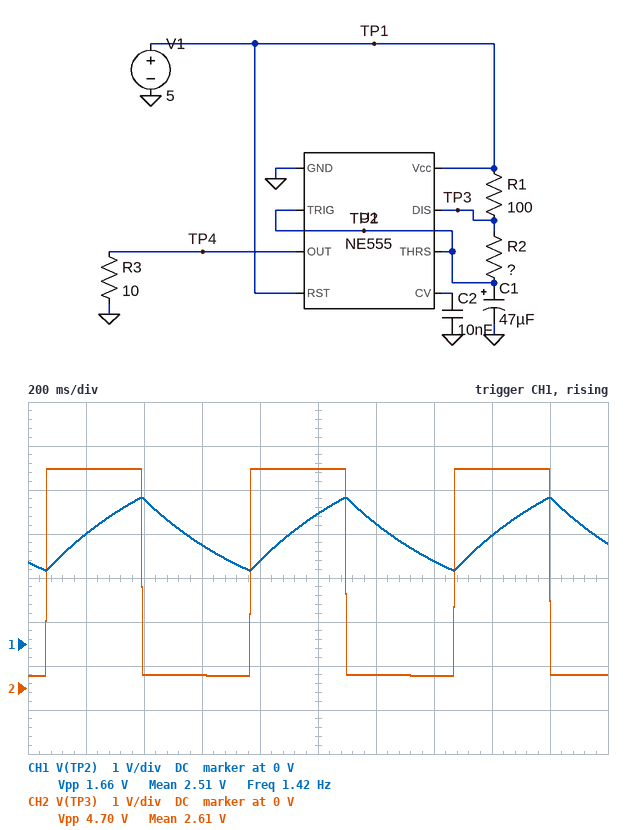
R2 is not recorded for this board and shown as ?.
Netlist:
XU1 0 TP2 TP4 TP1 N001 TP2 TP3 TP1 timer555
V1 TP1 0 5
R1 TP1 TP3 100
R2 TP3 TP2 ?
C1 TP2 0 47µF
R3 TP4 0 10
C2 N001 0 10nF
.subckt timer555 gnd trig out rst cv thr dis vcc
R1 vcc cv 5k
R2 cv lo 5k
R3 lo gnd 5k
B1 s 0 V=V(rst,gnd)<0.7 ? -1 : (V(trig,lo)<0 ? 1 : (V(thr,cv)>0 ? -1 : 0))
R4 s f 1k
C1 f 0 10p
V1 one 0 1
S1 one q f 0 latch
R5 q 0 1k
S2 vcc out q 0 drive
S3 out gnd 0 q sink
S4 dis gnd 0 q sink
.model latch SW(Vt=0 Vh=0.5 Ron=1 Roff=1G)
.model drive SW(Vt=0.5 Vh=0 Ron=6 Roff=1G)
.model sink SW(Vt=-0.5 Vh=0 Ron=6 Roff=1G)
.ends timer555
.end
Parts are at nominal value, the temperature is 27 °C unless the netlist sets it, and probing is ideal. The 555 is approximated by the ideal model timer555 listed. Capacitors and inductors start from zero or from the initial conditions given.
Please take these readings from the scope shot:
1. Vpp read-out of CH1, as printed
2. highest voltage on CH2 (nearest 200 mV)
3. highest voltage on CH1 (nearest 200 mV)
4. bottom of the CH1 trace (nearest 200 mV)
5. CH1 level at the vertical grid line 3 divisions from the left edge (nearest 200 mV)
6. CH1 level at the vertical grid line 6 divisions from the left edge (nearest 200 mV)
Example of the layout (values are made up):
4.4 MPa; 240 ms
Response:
1.66 V; 5.0 V; 3.4 V; 1.6 V; 2.2 V; 2.8 V
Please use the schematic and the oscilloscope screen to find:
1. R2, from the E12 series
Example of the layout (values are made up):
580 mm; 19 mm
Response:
10 kΩ
